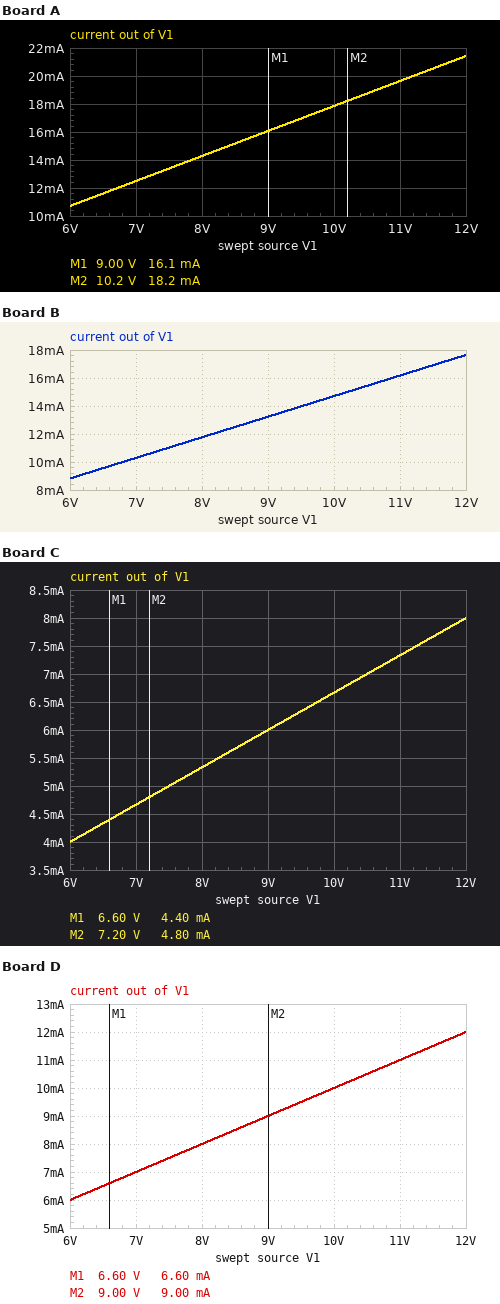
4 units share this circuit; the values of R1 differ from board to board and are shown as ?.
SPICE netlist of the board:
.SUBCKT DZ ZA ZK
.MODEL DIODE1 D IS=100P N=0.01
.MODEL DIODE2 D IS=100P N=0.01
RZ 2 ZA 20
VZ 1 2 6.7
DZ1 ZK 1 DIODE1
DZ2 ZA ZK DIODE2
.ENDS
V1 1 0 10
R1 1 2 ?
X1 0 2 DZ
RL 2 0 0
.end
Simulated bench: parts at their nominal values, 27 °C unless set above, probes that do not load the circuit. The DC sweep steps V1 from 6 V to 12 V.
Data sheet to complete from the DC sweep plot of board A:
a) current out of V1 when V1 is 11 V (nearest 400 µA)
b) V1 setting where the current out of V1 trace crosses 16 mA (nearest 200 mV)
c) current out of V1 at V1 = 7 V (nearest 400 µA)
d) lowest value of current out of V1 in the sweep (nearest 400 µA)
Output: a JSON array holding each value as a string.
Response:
["19.6 mA", "9.0 V", "12.4 mA", "10.8 mA"]
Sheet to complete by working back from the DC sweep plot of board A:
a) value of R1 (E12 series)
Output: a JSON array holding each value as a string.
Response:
["560 Ω"]
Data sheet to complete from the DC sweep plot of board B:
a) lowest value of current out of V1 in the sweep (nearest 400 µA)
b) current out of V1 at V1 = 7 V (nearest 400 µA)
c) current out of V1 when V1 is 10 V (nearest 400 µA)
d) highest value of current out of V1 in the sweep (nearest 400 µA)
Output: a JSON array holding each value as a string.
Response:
["8.8 mA", "10.4 mA", "14.8 mA", "17.6 mA"]
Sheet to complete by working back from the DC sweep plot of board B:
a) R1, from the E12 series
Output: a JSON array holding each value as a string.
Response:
["680 Ω"]
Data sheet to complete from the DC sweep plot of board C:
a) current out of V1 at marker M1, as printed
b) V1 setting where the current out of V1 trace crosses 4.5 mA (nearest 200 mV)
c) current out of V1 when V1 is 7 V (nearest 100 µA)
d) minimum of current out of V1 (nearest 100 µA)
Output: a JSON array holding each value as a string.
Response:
["4.40 mA", "6.8 V", "4.7 mA", "4.0 mA"]
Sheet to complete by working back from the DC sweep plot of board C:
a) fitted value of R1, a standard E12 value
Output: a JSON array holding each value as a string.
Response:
["1.5 kΩ"]
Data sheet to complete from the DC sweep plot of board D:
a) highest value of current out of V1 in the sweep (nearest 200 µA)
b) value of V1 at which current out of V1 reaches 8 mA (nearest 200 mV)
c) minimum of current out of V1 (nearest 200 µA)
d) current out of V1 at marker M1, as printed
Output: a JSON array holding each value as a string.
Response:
["12.0 mA", "8.0 V", "6.0 mA", "6.60 mA"]
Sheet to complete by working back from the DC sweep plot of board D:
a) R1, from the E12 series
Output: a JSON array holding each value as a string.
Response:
["1 kΩ"]
